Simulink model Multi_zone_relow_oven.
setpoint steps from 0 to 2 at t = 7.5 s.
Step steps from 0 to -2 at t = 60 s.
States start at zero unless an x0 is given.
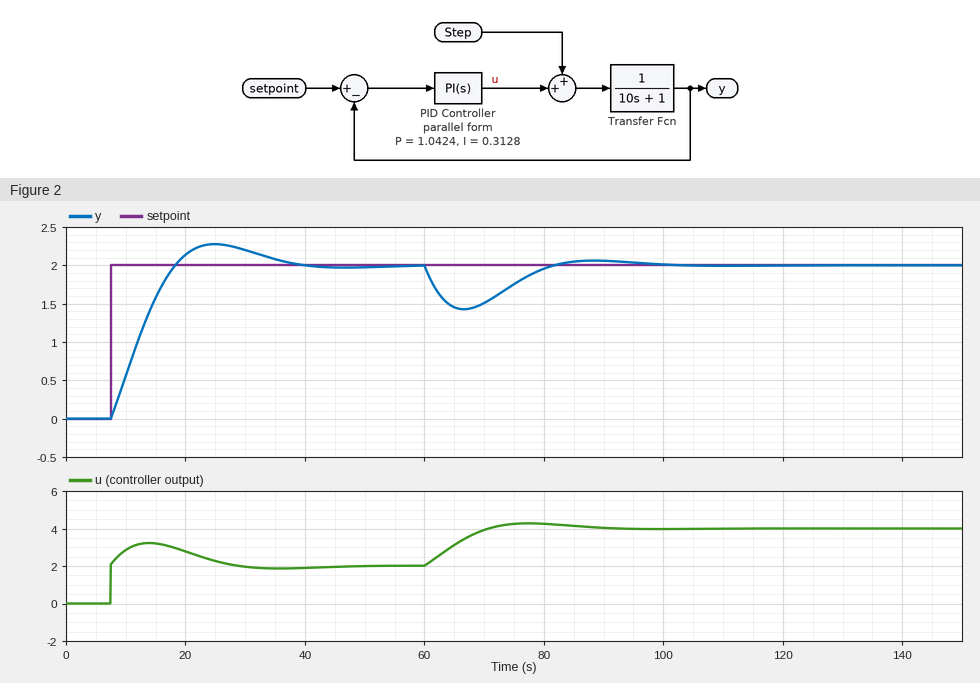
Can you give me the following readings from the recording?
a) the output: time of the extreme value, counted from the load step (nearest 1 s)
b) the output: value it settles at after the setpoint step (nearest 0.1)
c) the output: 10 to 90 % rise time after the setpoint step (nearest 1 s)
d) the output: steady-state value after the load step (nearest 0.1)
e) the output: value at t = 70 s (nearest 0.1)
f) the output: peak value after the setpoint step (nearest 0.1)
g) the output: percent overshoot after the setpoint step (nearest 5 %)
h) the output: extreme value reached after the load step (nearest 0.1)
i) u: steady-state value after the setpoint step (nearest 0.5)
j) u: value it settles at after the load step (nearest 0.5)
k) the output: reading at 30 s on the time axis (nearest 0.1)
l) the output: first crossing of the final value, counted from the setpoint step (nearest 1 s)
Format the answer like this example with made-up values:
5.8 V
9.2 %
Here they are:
7 s
2.0
8 s
2.0
1.5
2.3
15 %
1.4
2.0
4.0
2.2
11 s
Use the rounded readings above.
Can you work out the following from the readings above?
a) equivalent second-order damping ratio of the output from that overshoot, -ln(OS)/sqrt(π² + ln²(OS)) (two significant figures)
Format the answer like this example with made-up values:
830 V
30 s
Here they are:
0.52
